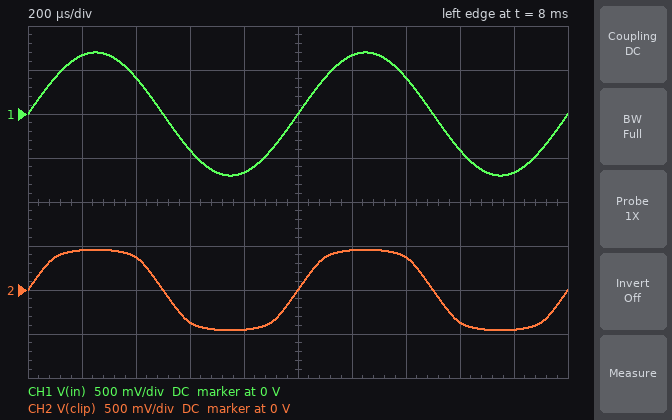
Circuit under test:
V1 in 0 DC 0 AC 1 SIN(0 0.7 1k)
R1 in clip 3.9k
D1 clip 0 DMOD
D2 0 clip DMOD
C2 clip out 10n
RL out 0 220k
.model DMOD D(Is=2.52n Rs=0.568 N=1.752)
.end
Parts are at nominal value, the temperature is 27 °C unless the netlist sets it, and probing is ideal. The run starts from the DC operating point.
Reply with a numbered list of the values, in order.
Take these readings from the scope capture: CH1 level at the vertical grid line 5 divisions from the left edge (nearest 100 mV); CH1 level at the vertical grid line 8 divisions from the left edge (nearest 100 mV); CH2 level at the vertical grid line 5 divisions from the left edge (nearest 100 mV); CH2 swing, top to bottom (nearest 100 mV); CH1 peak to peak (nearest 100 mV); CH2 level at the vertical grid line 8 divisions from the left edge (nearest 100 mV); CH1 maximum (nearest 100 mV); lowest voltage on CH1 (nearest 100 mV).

1. 0 V
2. -400 mV
3. 0 V
4. 900 mV
5. 1.4 V
6. -400 mV
7. 700 mV
8. -700 mV
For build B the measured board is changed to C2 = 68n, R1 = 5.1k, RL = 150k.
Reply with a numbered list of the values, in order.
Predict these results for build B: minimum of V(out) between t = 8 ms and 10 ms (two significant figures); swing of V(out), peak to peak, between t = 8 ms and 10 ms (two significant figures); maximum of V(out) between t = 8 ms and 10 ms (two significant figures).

1. -450 mV
2. 890 mV
3. 440 mV
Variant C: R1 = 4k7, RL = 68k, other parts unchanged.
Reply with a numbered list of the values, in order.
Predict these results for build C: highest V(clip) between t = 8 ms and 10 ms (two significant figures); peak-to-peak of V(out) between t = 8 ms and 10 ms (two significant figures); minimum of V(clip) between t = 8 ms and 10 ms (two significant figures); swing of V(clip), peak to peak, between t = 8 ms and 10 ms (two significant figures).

1. 450 mV
2. 920 mV
3. -450 mV
4. 890 mV
